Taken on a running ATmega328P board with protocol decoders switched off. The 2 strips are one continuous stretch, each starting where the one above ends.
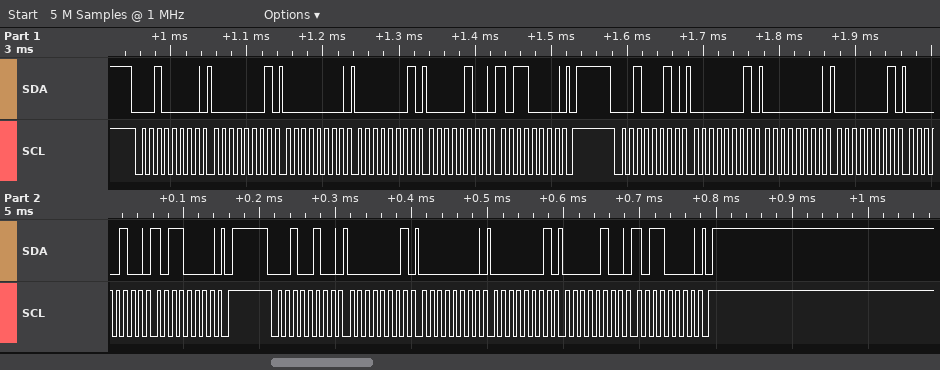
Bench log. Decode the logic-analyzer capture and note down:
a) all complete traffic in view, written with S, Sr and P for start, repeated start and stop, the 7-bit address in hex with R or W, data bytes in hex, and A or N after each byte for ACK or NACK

S 10W A 01 A 00 A 01 A 04 A B0 A P S 11W A 01 A 00 A 01 A 04 A B0 A P S 12W A 01 A 00 A 01 A 04 A B0 A P
